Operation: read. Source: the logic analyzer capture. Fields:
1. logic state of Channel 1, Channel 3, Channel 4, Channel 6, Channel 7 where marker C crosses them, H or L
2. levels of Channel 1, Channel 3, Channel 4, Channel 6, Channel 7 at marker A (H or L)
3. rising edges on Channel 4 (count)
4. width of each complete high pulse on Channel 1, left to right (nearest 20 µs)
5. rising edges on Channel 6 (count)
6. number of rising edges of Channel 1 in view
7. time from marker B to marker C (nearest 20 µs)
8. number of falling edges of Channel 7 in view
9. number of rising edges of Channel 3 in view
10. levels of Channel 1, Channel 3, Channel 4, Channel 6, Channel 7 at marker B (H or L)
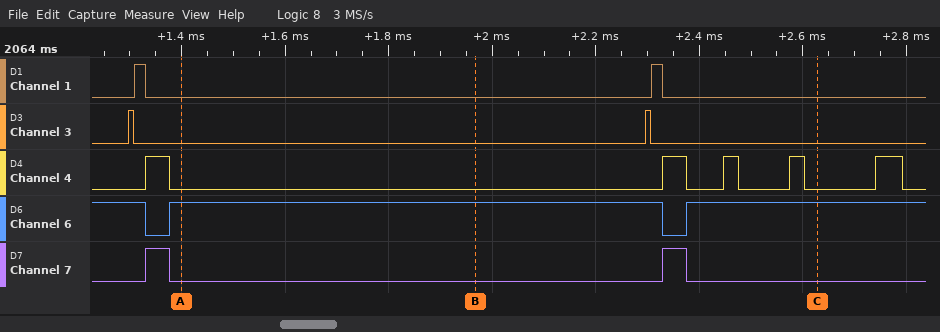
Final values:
Channel 1=L, Channel 3=L, Channel 4=L, Channel 6=H, Channel 7=L
Channel 1=L, Channel 3=L, Channel 4=L, Channel 6=H, Channel 7=L
5
20 µs, 20 µs
2
2
660 µs
2
2
Channel 1=L, Channel 3=L, Channel 4=L, Channel 6=H, Channel 7=L
